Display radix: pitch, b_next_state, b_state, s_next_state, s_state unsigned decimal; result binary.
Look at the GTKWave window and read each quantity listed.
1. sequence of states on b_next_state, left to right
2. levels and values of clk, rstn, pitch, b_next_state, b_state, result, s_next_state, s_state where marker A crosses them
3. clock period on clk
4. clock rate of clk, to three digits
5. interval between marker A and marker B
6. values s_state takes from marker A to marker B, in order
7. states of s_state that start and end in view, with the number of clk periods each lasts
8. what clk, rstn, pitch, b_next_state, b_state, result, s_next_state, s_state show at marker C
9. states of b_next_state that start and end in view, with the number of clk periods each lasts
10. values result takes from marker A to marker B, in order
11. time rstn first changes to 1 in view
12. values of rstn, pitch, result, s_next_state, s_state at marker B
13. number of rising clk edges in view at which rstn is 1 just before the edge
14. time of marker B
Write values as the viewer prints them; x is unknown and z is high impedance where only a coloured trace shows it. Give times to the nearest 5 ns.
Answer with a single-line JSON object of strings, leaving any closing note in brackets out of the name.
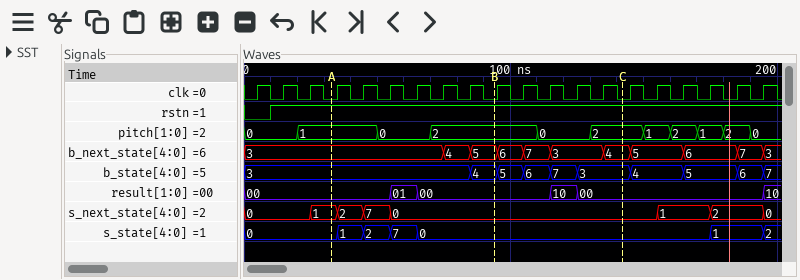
{"sequence of states on b_next_state, left to right": "3, 4, 5, 6, 7, 3, 4, 5, 6, 7, 3", "levels and values of clk, rstn, pitch, b_next_state, b_state, result, s_next_state, s_state where marker A crosses them": "clk=0, rstn=1, pitch=1, b_next_state=3, b_state=3, result=00, s_next_state=1, s_state=0", "clock period on clk": "10 ns", "clock rate of clk, to three digits": "100 MHz", "interval between marker A and marker B": "60 ns", "values s_state takes from marker A to marker B, in order": "0, 1, 2, 7, 0", "states of s_state that start and end in view, with the number of clk periods each lasts": "1: 1, 2: 1, 7: 1, 0: 11, 1: 2", "what clk, rstn, pitch, b_next_state, b_state, result, s_next_state, s_state show at marker C": "clk=0, rstn=1, pitch=2, b_next_state=4, b_state=3, result=00, s_next_state=0, s_state=0", "states of b_next_state that start and end in view, with the number of clk periods each lasts": "4: 1, 5: 1, 6: 1, 7: 1, 3: 2, 4: 1, 5: 2, 6: 2, 7: 1", "values result takes from marker A to marker B, in order": "00, 01, 00", "time rstn first changes to 1 in view": "10 ns", "values of rstn, pitch, result, s_next_state, s_state at marker B": "rstn=1, pitch=2, result=00, s_next_state=0, s_state=0", "number of rising clk edges in view at which rstn is 1 just before the edge": "19", "time of marker B": "95 ns"}
